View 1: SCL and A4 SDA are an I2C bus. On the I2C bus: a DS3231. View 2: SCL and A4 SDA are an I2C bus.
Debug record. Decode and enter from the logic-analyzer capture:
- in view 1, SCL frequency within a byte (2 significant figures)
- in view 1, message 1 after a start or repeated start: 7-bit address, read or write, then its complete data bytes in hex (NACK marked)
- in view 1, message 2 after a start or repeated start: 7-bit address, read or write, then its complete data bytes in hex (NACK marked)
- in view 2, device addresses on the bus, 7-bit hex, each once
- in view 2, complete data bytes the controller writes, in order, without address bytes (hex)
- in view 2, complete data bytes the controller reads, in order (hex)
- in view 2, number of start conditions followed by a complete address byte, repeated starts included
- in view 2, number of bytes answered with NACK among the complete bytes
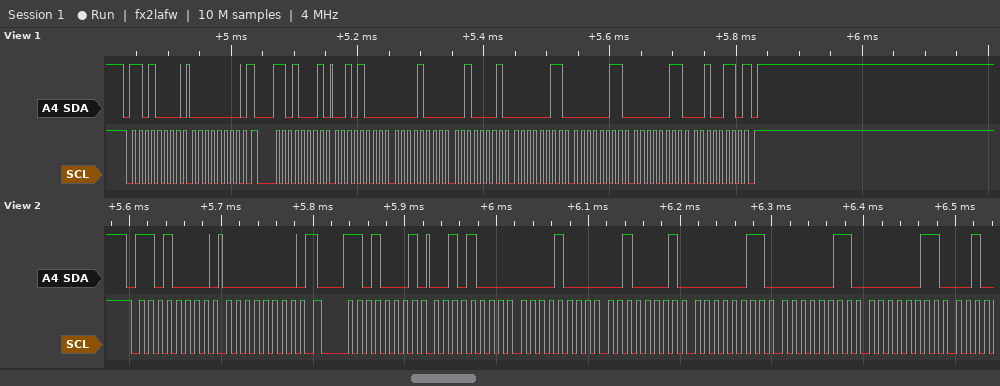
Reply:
100 kHz
0x68 write: 00
0x68 read: 28 08 21 03 03 03 26 NACK
0x68
00
28 08 21 03 03 03
2
0
